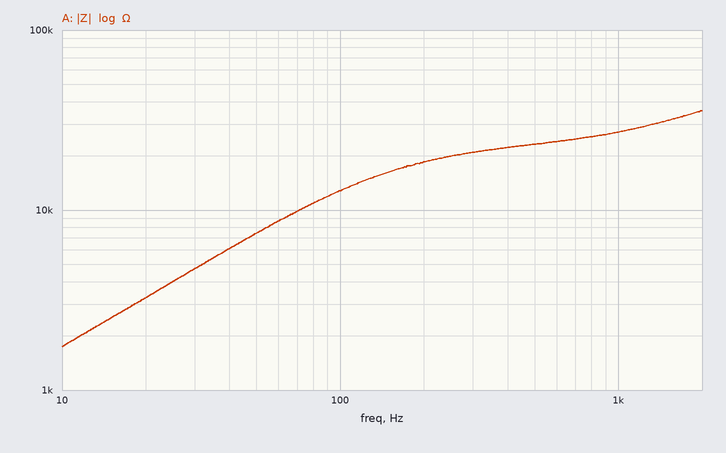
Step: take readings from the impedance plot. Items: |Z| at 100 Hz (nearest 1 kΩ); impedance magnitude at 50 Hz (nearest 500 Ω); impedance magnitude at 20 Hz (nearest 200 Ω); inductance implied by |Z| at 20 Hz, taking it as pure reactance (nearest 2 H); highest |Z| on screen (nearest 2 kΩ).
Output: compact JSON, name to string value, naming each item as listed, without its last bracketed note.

{"|Z| at 100 Hz": "13 kΩ", "impedance magnitude at 50 Hz": "7.5 kΩ", "impedance magnitude at 20 Hz": "3.2 kΩ", "inductance implied by |Z| at 20 Hz, taking it as pure reactance": "26 H", "highest |Z| on screen": "36 kΩ"}
